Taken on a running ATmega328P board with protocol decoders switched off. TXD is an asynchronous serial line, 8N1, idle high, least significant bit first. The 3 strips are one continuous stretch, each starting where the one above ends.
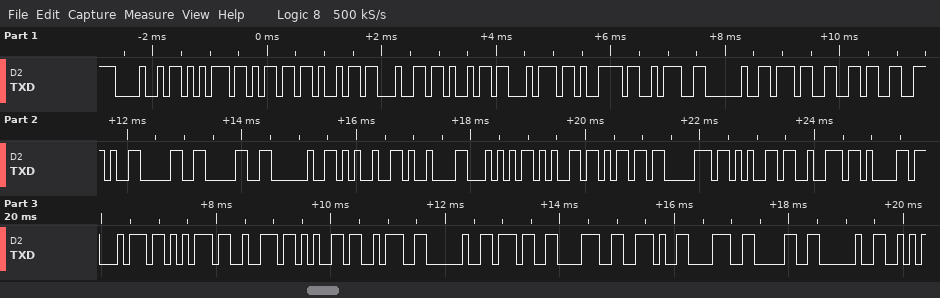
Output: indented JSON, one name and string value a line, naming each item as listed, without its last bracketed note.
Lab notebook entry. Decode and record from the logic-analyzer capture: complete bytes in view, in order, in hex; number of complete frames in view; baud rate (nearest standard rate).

{
  "complete bytes in view, in order, in hex": "48 75 6D 69 64 69 74 79 3A 20 37 36 2E 30 30 20 25 09 54 65 6D 70 65 72 61 74 75 72 65 3A 20 37 38 2E 38 30 20",
  "number of complete frames in view": "37",
  "baud rate": "9600 baud"
}
